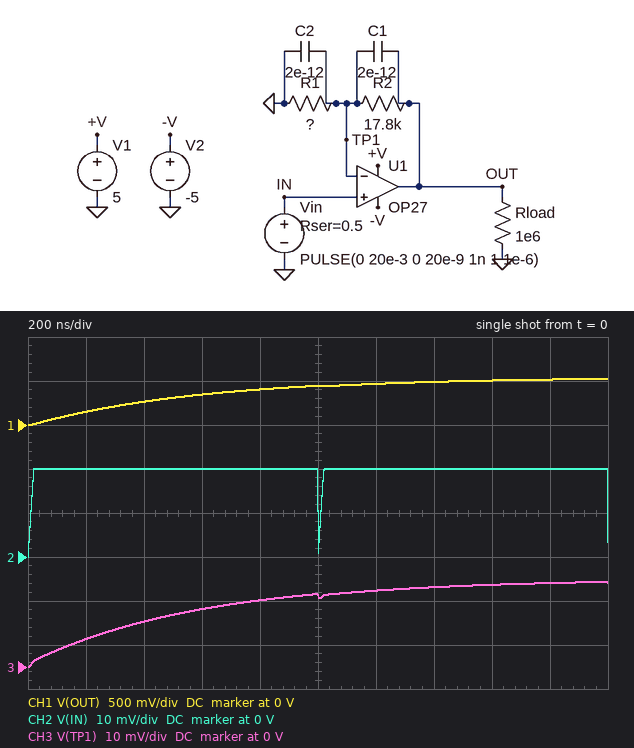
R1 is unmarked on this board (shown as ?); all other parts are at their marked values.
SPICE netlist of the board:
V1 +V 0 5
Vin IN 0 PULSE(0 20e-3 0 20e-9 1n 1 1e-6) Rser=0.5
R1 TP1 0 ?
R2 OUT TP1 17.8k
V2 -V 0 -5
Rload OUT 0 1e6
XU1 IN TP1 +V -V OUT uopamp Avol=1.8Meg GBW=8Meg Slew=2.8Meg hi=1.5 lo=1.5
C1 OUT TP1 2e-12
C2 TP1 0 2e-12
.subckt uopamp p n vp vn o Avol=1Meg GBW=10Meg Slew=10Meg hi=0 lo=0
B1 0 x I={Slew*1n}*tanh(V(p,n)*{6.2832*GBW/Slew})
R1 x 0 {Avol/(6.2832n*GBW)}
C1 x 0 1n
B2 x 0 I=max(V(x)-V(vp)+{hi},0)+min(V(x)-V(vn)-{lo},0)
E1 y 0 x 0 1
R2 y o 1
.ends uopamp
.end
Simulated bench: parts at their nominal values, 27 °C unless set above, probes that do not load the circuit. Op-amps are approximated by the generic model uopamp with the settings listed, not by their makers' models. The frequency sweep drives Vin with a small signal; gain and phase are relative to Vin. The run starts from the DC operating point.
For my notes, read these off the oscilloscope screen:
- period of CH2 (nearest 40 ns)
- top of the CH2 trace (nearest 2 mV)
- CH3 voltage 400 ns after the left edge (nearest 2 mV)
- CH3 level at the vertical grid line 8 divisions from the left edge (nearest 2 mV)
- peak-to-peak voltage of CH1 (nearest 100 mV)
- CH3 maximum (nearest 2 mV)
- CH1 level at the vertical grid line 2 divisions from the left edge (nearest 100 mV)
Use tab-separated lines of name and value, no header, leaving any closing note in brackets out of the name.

period of CH2	1.00 µs
top of the CH2 trace	20 mV
CH3 voltage 400 ns after the left edge	10 mV
CH3 level at the vertical grid line 8 divisions from the left edge	18 mV
peak-to-peak voltage of CH1	500 mV
CH3 maximum	20 mV
CH1 level at the vertical grid line 2 divisions from the left edge	300 mV
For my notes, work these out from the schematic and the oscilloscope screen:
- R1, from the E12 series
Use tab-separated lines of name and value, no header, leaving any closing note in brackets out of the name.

R1, from the E12 series	680 Ω
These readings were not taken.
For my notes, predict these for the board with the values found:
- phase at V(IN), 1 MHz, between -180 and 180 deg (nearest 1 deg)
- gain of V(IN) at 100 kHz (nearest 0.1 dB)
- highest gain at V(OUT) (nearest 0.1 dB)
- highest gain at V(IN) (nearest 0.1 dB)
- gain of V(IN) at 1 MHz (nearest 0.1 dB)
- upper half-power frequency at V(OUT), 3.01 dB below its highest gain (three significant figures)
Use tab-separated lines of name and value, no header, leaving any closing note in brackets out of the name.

phase at V(IN), 1 MHz, between -180 and 180 deg	0 deg
gain of V(IN) at 100 kHz	0 dB
highest gain at V(OUT)	28.7 dB
highest gain at V(IN)	0 dB
gain of V(IN) at 1 MHz	0 dB
upper half-power frequency at V(OUT), 3.01 dB below its highest gain	277 kHz
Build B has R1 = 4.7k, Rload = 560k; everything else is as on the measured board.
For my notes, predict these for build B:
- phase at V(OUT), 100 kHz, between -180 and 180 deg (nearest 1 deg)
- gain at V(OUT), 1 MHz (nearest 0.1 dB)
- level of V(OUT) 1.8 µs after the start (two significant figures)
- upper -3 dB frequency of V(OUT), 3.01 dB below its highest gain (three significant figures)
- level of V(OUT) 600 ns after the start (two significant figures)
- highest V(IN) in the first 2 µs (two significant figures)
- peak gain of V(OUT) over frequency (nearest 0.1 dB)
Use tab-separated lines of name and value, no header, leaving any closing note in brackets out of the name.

phase at V(OUT), 100 kHz, between -180 and 180 deg	-4 deg
gain at V(OUT), 1 MHz	11.7 dB
level of V(OUT) 1.8 µs after the start	96 mV
upper -3 dB frequency of V(OUT), 3.01 dB below its highest gain	1.35 MHz
level of V(OUT) 600 ns after the start	95 mV
highest V(IN) in the first 2 µs	20 mV
peak gain of V(OUT) over frequency	13.6 dB
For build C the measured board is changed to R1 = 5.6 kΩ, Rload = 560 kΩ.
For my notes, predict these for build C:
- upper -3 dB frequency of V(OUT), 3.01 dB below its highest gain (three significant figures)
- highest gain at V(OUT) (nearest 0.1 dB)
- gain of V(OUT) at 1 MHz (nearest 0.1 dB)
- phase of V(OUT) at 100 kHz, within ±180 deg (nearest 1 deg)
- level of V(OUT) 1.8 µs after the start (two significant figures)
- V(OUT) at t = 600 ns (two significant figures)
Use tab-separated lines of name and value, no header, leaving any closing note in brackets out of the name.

upper -3 dB frequency of V(OUT), 3.01 dB below its highest gain	1.53 MHz
highest gain at V(OUT)	12.4 dB
gain of V(OUT) at 1 MHz	10.9 dB
phase of V(OUT) at 100 kHz, within ±180 deg	-4 deg
level of V(OUT) 1.8 µs after the start	84 mV
V(OUT) at t = 600 ns	83 mV
